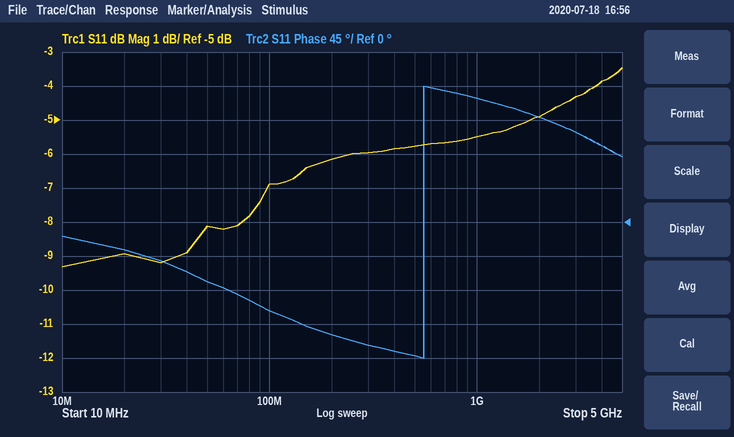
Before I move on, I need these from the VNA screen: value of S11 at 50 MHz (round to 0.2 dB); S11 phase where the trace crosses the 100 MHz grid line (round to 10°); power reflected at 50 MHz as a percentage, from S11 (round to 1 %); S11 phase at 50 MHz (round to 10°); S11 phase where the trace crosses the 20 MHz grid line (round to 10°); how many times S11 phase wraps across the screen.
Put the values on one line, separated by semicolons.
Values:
-8.2 dB; -120°; 15 %; -80°; -40°; 1
